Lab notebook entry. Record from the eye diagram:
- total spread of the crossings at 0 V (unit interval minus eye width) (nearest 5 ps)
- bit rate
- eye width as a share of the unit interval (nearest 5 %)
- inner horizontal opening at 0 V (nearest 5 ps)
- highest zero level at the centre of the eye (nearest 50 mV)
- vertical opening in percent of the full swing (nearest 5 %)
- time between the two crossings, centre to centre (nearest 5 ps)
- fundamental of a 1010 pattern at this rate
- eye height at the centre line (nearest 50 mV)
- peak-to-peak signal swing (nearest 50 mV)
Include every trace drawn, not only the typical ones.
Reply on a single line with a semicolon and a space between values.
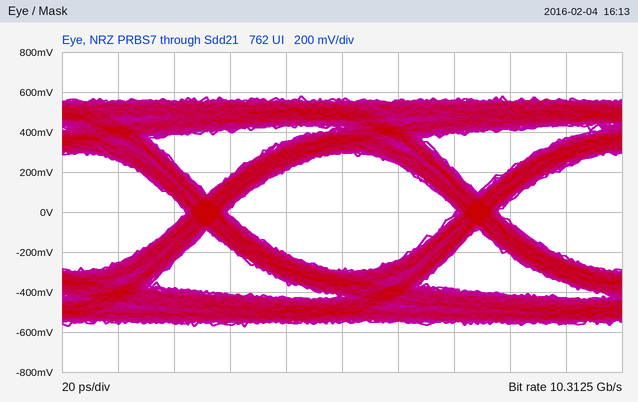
15 ps; 10.3125 Gb/s; 85 %; 80 ps; -300 mV; 50 %; 95 ps; 5.15625 GHz; 600 mV; 1.15 V
